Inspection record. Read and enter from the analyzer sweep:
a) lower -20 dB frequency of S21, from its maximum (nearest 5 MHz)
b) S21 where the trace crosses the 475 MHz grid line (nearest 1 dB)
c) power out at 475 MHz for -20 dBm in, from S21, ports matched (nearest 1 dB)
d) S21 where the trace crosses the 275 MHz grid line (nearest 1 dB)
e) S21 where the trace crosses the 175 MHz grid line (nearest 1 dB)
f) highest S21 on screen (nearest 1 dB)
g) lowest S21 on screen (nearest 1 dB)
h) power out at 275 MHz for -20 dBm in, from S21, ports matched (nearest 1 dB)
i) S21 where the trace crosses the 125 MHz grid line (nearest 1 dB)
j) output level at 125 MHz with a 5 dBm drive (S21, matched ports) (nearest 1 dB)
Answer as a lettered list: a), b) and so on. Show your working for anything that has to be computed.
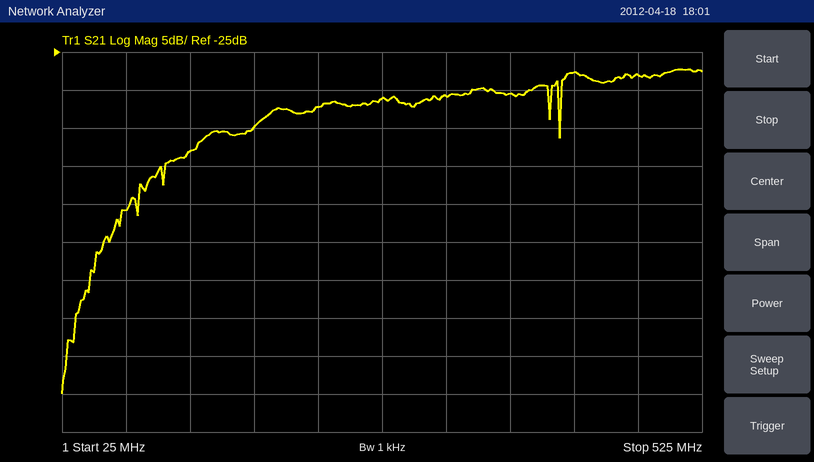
a) 70 MHz
b) -28 dB
c) -20 dBm + (-28 dB) = -48 dBm
d) -31 dB
e) -35 dB
f) -27 dB
g) -70 dB
h) -20 dBm + (-31 dB) = -51 dBm
i) -38 dB
j) 5 dBm + (-38 dB) = -33 dBm
